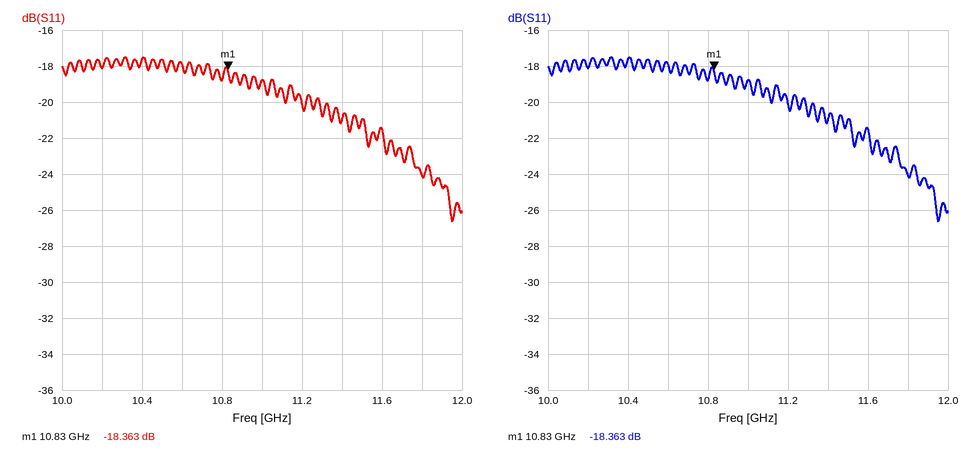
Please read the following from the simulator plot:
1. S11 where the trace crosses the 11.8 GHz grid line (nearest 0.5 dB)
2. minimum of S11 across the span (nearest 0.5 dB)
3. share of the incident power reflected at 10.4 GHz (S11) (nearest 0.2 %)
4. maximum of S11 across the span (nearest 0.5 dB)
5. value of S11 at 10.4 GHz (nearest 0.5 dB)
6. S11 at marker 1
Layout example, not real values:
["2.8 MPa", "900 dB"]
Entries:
["-24.0 dB", "-26.5 dB", "1.8 %", "-17.5 dB", "-17.5 dB", "-18.363 dB"]
